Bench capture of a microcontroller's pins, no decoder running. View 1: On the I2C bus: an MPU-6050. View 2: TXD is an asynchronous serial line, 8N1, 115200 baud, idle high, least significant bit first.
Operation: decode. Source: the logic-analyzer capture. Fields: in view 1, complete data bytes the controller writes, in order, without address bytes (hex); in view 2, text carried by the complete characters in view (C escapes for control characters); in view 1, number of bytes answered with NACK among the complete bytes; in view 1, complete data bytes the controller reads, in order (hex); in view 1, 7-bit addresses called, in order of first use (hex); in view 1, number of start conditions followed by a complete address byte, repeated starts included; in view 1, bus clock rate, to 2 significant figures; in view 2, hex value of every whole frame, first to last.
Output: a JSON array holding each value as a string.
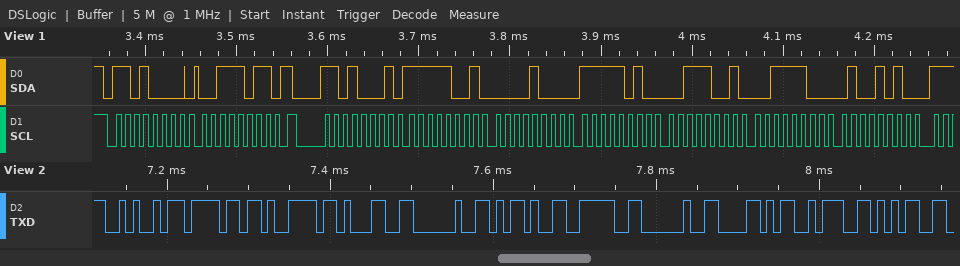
["3B", "\"Joy1 -> X:5\"", "0", "F9 08 FA 39 3C 4A", "0x68", "2", "100 kHz", "4A 6F 79 31 20 2D 3E 20 58 3A 35"]
